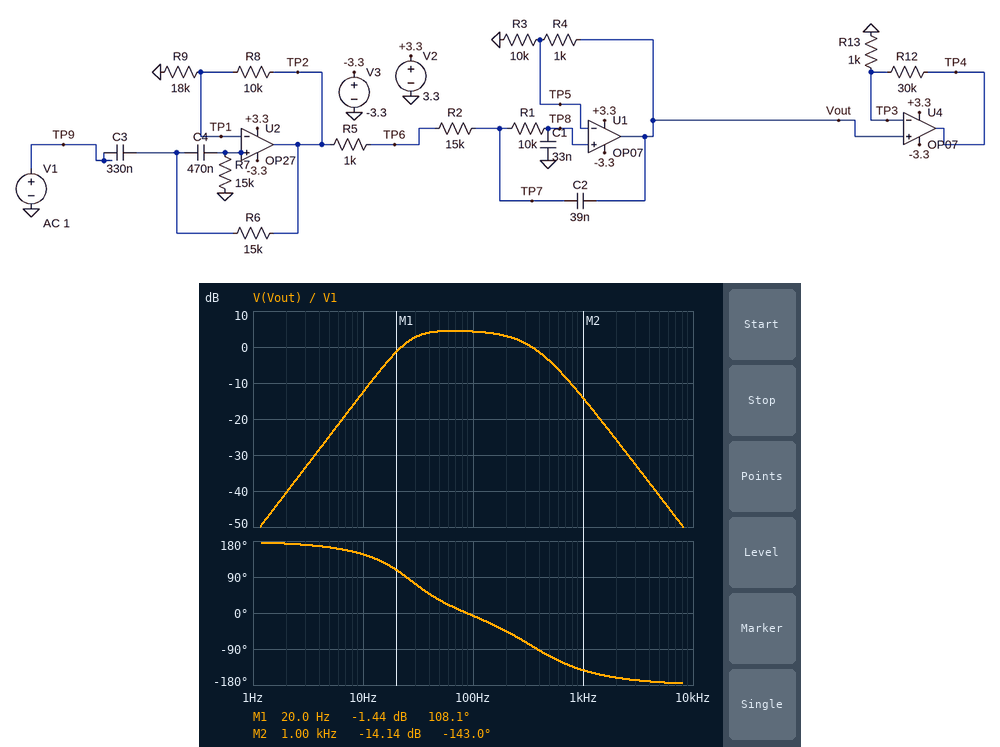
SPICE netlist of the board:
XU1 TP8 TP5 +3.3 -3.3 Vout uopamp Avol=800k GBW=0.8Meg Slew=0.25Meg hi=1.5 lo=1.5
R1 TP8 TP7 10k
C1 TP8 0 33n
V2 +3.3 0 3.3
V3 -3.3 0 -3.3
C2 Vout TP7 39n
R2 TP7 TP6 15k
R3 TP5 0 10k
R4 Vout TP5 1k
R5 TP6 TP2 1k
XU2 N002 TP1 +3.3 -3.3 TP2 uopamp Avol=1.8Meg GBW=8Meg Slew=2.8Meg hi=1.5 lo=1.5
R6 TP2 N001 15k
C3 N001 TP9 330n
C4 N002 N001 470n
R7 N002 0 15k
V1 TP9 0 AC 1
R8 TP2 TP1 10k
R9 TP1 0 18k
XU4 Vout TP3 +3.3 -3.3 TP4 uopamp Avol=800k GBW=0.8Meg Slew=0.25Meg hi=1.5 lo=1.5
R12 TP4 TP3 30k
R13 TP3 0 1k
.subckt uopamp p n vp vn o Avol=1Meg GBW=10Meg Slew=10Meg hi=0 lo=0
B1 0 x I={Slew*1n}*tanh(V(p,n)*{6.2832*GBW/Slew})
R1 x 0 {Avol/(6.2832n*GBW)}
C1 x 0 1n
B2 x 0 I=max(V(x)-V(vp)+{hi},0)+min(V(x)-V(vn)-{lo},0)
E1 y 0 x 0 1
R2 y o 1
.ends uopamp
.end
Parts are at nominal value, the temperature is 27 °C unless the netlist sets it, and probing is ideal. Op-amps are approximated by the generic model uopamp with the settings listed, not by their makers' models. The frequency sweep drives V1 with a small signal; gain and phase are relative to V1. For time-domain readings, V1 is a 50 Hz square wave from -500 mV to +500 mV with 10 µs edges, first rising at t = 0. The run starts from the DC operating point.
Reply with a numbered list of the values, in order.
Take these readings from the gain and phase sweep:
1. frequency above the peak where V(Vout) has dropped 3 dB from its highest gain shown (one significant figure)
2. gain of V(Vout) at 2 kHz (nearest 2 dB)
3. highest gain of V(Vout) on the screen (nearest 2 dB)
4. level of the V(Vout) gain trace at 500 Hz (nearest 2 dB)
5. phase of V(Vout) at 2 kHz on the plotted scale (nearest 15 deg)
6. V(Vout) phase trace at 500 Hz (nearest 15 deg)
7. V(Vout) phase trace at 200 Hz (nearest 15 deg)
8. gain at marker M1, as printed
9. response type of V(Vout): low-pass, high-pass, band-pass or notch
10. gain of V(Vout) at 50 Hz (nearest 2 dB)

1. 300 Hz
2. -26 dB
3. 4 dB
4. -4 dB
5. -165 deg
6. -105 deg
7. -45 deg
8. -1.44 dB
9. band-pass
10. 4 dB
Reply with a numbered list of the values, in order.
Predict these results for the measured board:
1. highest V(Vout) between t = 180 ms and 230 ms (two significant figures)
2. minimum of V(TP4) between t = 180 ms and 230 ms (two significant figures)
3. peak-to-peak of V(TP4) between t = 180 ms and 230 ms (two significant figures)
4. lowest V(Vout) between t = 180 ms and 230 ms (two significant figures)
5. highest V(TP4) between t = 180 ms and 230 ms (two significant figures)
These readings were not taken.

1. 1.4 V
2. -1.8 V
3. 3.6 V
4. -1.4 V
5. 1.8 V
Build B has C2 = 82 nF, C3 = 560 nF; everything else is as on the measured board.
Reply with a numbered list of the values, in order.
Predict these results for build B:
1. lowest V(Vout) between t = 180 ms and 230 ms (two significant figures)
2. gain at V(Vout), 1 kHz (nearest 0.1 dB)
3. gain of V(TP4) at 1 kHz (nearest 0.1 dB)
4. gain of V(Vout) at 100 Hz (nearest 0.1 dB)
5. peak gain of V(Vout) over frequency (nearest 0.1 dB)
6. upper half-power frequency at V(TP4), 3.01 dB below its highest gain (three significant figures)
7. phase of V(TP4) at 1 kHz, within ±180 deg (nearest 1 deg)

1. -1.5 V
2. -19.8 dB
3. 10.0 dB
4. 5.1 dB
5. 5.4 dB
6. 277 Hz
7. -165 deg
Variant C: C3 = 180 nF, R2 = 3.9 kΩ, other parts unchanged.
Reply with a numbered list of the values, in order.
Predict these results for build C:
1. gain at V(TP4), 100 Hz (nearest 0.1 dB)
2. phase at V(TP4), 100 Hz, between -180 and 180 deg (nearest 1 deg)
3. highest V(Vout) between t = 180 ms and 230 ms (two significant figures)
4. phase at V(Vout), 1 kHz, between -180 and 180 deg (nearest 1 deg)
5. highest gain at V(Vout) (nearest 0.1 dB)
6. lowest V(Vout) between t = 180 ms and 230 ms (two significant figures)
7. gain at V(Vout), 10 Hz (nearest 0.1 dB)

1. 34.4 dB
2. 12 deg
3. 1.6 V
4. -114 deg
5. 4.6 dB
6. -1.6 V
7. -17.8 dB
